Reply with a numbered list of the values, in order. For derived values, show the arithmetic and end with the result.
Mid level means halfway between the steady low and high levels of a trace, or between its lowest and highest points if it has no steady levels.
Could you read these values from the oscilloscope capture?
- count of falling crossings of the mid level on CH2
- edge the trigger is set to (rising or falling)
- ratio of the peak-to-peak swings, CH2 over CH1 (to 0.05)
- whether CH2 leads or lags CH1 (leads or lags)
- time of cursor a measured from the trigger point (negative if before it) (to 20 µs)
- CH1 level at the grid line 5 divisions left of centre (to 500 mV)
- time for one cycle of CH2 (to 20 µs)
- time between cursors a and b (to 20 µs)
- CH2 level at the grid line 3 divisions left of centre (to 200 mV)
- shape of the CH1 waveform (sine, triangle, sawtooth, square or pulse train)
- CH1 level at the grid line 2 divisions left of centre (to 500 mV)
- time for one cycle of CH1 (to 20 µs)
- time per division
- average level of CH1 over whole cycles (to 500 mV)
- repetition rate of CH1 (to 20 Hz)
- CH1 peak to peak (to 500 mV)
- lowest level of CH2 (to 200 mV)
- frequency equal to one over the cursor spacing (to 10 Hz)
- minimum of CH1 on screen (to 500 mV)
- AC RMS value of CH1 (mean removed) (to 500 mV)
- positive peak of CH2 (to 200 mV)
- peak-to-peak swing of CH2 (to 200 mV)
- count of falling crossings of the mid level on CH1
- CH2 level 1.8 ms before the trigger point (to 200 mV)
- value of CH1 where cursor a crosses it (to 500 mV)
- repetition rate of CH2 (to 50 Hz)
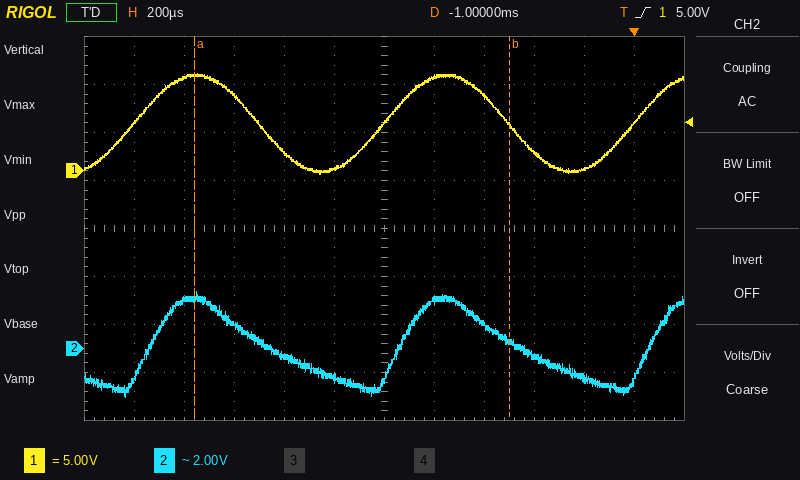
1. 2
2. rising
3. 4.4 V / 10.5 V ≈ 0.419, so 0.40 to the nearest 0.05
4. lags
5. -1.76 ms
6. 5.0 V
7. 1.00 ms
8. 1.26 ms
9. 1.0 V
10. sine
11. 2.0 V
12. 1.00 ms
13. 200 µs
14. (10.0 V + (-500 mV)) / 2 ≈ 4.75 V, so 5.0 V to the nearest 500 mV
15. 1 / 1.00 ms ≈ 1.00 kHz
16. 10.0 V − (-500 mV) = 10.5 V
17. -2.0 V
18. 1 / 1.26 ms ≈ 790 Hz
19. -500 mV
20. 10.5 V / (2√2) ≈ 3.71 V, so 3.5 V to the nearest 500 mV
21. 2.4 V
22. 2.4 V − (-2.0 V) = 4.4 V
23. 2
24. 2.0 V
25. 10.0 V
26. 1 / 1.00 ms ≈ 1.00 kHz
